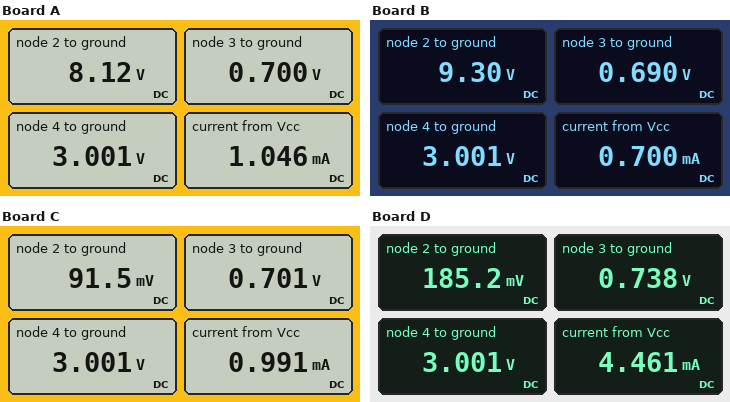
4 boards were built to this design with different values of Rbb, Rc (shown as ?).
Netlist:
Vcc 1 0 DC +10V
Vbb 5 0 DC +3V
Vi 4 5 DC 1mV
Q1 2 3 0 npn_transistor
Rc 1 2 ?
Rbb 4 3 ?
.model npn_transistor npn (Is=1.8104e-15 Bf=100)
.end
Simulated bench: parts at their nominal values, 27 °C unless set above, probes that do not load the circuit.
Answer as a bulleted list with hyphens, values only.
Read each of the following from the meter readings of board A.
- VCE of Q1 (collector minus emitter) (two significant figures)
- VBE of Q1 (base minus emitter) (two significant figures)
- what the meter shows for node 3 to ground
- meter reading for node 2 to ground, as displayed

- 8.1 V
- 700 mV
- 0.700 V
- 8.12 V
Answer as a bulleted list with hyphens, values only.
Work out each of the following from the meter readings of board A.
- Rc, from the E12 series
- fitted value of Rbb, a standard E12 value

- 1.8 kΩ
- 220 kΩ
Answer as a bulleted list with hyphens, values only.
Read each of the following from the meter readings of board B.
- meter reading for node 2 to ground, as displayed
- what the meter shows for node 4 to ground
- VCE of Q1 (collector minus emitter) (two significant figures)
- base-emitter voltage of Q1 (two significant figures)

- 9.30 V
- 3.001 V
- 9.3 V
- 690 mV
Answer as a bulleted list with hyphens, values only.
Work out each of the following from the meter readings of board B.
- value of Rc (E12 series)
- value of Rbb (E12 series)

- 1 kΩ
- 330 kΩ
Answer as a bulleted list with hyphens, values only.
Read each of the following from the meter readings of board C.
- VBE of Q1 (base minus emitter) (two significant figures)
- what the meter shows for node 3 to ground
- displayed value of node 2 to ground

- 700 mV
- 0.701 V
- 91.5 mV
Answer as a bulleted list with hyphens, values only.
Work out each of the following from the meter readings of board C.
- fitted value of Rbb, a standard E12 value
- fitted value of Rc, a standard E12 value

- 56 kΩ
- 10 kΩ
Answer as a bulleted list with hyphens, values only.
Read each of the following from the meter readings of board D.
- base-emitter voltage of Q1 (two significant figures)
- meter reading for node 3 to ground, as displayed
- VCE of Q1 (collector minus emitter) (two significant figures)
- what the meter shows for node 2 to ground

- 740 mV
- 0.738 V
- 190 mV
- 185.2 mV
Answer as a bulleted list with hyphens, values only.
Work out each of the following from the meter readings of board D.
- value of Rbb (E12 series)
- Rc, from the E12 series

- 47 kΩ
- 2.2 kΩ
